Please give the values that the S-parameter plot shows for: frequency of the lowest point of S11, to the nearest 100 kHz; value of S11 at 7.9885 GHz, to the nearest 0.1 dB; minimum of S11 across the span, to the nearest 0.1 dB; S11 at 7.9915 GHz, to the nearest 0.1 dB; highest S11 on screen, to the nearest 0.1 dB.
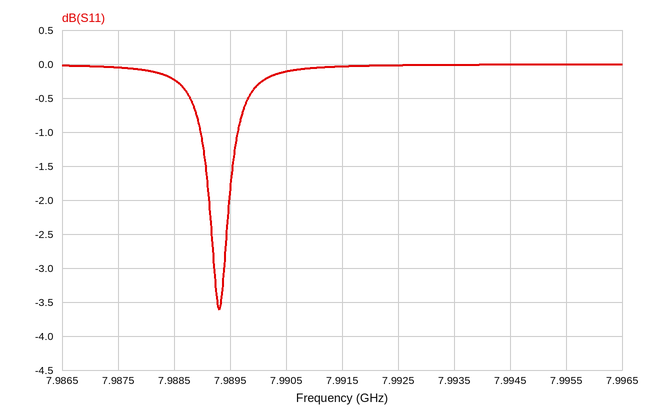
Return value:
7.9893 GHz
-0.2 dB
-3.6 dB
0.0 dB
0.0 dB
